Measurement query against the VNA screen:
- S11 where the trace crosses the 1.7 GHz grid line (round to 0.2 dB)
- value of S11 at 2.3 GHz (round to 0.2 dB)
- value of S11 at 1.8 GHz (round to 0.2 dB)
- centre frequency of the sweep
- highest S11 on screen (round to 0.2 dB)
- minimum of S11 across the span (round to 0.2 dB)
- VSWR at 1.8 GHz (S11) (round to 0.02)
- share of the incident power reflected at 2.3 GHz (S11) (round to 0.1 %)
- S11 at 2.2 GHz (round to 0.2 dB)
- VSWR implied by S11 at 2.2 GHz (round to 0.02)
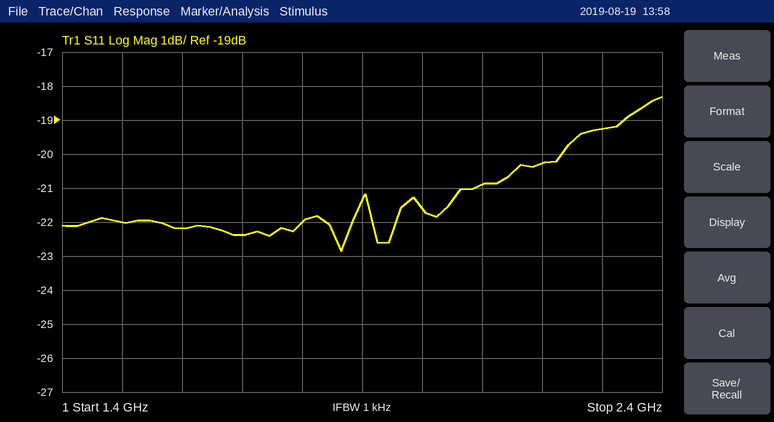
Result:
-22.4 dB
-19.2 dB
-22.0 dB
1.9 GHz
-18.4 dB
-22.8 dB
1.18
1.2 %
-20.2 dB
1.22
